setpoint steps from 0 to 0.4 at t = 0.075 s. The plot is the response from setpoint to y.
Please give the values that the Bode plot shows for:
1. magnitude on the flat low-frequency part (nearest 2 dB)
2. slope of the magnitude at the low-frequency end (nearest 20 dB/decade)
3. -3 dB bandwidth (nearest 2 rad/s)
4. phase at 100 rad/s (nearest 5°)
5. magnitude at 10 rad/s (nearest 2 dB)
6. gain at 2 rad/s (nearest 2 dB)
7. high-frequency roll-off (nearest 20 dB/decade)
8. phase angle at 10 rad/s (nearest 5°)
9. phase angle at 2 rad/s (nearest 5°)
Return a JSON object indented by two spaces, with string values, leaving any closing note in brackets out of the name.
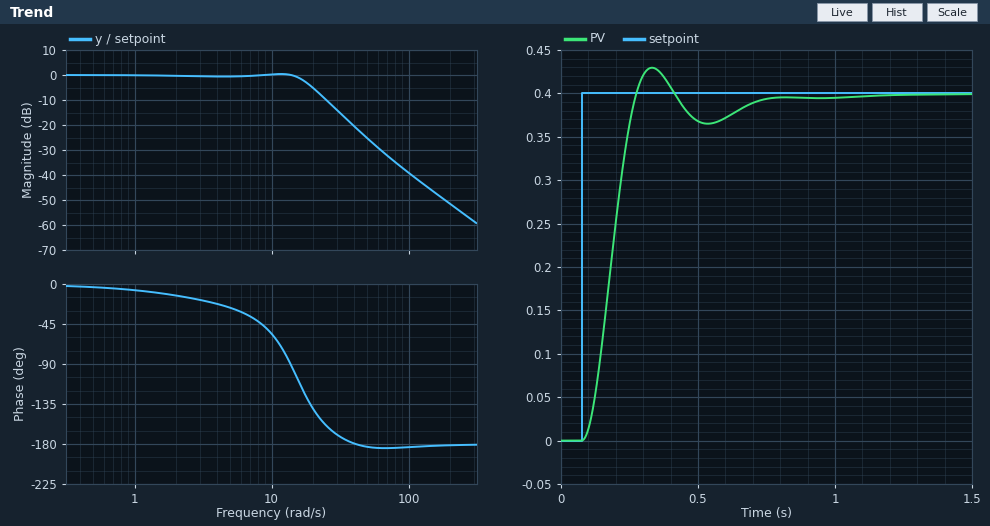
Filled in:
{
  "magnitude on the flat low-frequency part": "0 dB",
  "slope of the magnitude at the low-frequency end": "0 dB/decade",
  "-3 dB bandwidth": "18 rad/s",
  "phase at 100 rad/s": "-185°",
  "magnitude at 10 rad/s": "0 dB",
  "gain at 2 rad/s": "0 dB",
  "high-frequency roll-off": "-40 dB/decade",
  "phase angle at 10 rad/s": "-55°",
  "phase angle at 2 rad/s": "-15°"
}
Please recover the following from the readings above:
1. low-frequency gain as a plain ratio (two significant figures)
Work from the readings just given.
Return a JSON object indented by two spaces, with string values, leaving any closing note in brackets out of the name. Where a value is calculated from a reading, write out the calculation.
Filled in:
{
  "low-frequency gain as a plain ratio": "10^(0 / 20) = 1.0"
}
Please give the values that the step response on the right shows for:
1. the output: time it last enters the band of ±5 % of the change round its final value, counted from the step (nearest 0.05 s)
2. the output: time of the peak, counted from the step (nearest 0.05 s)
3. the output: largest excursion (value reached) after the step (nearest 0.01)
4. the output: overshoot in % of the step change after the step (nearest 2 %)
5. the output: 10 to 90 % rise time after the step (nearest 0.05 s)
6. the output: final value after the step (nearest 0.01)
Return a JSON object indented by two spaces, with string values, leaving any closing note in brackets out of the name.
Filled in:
{
  "the output: time it last enters the band of ±5 % of the change round its final value, counted from the step": "0.55 s",
  "the output: time of the peak, counted from the step": "0.25 s",
  "the output: largest excursion (value reached) after the step": "0.43",
  "the output: overshoot in % of the step change after the step": "8 %",
  "the output: 10 to 90 % rise time after the step": "0.15 s",
  "the output: final value after the step": "0.40"
}
